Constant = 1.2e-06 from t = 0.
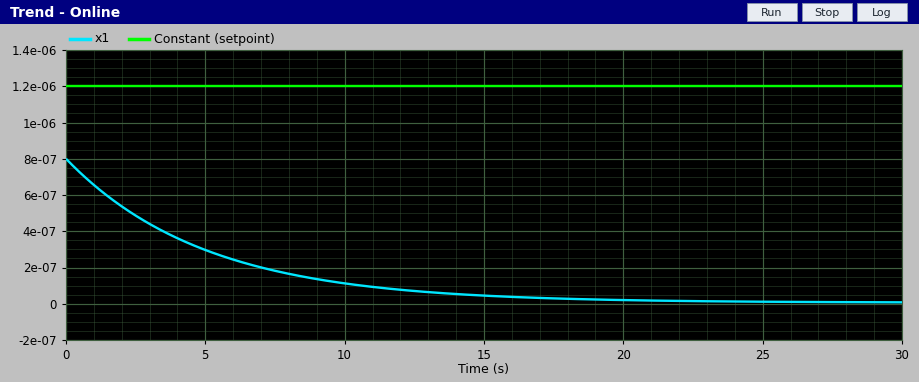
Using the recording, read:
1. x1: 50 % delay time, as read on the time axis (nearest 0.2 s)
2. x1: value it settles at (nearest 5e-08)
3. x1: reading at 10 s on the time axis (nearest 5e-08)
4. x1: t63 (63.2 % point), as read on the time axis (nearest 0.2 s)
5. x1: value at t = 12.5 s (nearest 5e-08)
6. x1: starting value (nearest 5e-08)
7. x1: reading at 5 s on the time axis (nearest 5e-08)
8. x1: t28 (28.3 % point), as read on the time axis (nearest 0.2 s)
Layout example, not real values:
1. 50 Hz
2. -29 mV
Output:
1. 3.4 s
2. 0.00000000
3. 0.00000010
4. 5.0 s
5. 0.00000005
6. 0.00000080
7. 0.00000030
8. 1.6 s
